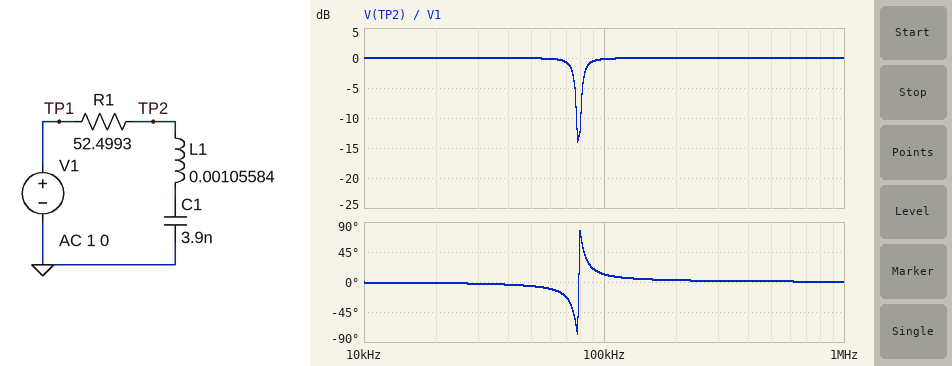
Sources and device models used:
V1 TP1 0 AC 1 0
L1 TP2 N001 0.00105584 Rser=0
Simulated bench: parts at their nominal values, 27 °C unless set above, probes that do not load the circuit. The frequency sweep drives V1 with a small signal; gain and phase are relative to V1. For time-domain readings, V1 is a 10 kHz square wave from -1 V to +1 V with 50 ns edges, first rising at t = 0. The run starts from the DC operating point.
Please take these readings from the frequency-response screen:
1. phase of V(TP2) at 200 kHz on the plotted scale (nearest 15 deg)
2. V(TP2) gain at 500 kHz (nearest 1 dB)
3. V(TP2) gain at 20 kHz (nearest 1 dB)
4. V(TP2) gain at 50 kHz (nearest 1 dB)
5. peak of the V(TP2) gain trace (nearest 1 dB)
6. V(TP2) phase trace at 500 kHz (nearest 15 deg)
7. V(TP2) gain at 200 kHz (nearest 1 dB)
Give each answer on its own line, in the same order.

0 deg
0 dB
0 dB
0 dB
0 dB
0 deg
0 dB
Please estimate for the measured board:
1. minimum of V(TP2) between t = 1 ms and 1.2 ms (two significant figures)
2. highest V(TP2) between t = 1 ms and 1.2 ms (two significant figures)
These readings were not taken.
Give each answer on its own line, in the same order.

-1.1 V
1.1 V
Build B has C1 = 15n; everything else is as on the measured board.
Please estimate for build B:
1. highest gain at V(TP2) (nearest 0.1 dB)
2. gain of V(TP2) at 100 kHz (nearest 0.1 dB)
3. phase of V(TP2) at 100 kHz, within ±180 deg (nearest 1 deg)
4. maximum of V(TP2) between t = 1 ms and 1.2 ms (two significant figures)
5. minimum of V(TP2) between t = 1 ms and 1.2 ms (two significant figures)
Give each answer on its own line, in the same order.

0 dB
0 dB
5 deg
1.2 V
-1.2 V
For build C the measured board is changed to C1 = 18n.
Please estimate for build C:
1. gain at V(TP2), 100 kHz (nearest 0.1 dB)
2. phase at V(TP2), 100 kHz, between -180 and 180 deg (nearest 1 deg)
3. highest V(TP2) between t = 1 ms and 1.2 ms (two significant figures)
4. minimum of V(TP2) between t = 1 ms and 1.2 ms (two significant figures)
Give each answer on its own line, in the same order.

0 dB
5 deg
1.2 V
-1.2 V
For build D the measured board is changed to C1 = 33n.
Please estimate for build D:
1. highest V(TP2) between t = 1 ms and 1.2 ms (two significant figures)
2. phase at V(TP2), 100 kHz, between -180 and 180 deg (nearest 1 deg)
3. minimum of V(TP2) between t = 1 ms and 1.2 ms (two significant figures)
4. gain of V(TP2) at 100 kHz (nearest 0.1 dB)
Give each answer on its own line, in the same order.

1.3 V
5 deg
-1.3 V
0 dB
